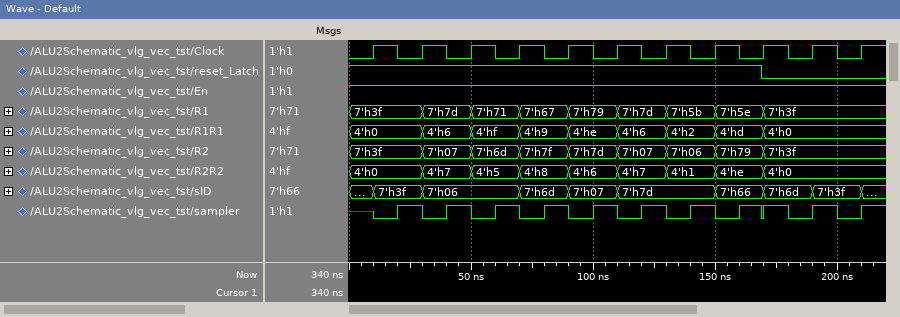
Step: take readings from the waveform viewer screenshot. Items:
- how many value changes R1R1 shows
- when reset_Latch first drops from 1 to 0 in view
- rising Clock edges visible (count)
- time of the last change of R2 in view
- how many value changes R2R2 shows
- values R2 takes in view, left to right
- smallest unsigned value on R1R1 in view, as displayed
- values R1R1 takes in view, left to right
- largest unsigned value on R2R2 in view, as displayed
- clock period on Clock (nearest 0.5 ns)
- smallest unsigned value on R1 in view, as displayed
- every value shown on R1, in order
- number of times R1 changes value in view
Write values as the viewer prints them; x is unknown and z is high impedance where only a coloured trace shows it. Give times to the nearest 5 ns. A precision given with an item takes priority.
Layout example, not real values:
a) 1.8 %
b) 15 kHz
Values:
a) 8
b) 170 ns
c) 11
d) 170 ns
e) 8
f) 7'h3f, 7'h07, 7'h6d, 7'h7f, 7'h7d, 7'h07, 7'h06, 7'h79, 7'h3f
g) 4'h0
h) 4'h0, 4'h6, 4'hf, 4'h9, 4'he, 4'h6, 4'h2, 4'hd, 4'h0
i) 4'he
j) 20 ns
k) 7'h3f
l) 7'h3f, 7'h7d, 7'h71, 7'h67, 7'h79, 7'h7d, 7'h5b, 7'h5e, 7'h3f
m) 8
